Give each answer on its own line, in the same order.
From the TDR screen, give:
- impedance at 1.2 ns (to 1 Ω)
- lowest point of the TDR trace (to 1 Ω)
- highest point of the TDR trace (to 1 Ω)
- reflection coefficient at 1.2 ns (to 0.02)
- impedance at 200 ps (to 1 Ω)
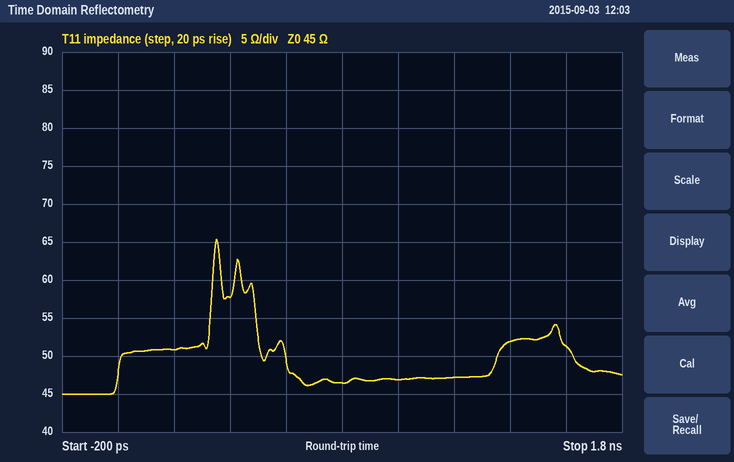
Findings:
47 Ω
45 Ω
65 Ω
+0.02
51 Ω
